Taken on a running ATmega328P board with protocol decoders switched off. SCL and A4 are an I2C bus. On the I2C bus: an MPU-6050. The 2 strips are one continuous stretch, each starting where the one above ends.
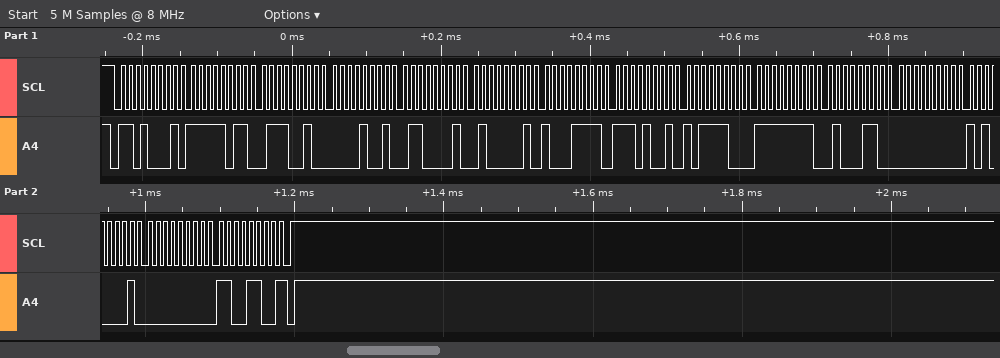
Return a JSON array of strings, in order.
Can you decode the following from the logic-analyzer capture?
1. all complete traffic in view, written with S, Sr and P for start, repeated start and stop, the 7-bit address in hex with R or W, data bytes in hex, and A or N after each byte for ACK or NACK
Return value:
["S 68R A FB A 72 A 09 A 61 A 41 A 8F A E9 A BC A FF A 46 A 00 A A1 A 00 A CC N P"]
